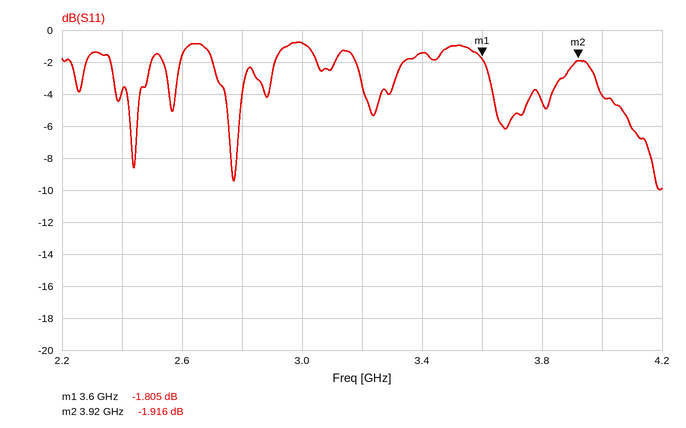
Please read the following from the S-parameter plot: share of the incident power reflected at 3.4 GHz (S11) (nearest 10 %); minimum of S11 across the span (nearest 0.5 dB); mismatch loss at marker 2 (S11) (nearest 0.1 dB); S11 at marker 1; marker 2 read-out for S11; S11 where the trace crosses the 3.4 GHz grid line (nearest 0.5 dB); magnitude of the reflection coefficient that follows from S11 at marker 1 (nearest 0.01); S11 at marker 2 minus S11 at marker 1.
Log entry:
70 %
-10.0 dB
4.5 dB
-1.805 dB
-1.916 dB
-1.5 dB
0.81
-0.111 dB
